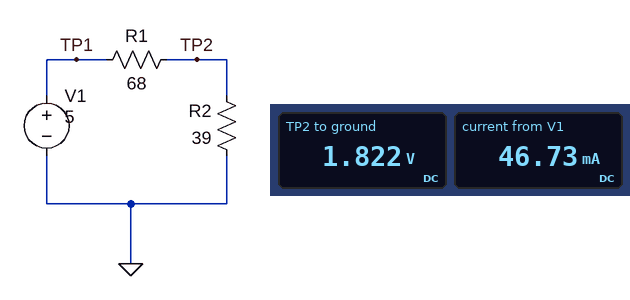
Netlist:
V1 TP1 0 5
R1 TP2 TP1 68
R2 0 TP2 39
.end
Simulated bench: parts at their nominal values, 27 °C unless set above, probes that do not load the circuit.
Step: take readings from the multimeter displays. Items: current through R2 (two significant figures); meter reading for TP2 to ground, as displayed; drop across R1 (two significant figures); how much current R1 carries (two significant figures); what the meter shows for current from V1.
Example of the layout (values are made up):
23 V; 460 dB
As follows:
47 mA; 1.822 V; 3.2 V; 47 mA; 46.73 mA
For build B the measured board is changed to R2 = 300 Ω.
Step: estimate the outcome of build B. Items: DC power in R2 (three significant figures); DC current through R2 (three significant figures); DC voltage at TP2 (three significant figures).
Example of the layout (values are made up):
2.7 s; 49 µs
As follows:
55.4 mW; 13.6 mA; 4.08 V
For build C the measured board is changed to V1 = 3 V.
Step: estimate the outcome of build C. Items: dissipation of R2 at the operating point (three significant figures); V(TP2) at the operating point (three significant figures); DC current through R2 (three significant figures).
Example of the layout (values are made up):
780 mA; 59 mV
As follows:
30.7 mW; 1.09 V; 28.0 mA
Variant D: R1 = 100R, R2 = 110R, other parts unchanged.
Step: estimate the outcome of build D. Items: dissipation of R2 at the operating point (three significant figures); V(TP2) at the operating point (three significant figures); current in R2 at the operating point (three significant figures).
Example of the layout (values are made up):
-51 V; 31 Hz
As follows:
62.4 mW; 2.62 V; 23.8 mA
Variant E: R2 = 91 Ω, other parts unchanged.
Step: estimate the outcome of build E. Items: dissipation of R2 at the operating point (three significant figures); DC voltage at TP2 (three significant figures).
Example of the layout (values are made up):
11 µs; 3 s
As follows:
90.0 mW; 2.86 V
